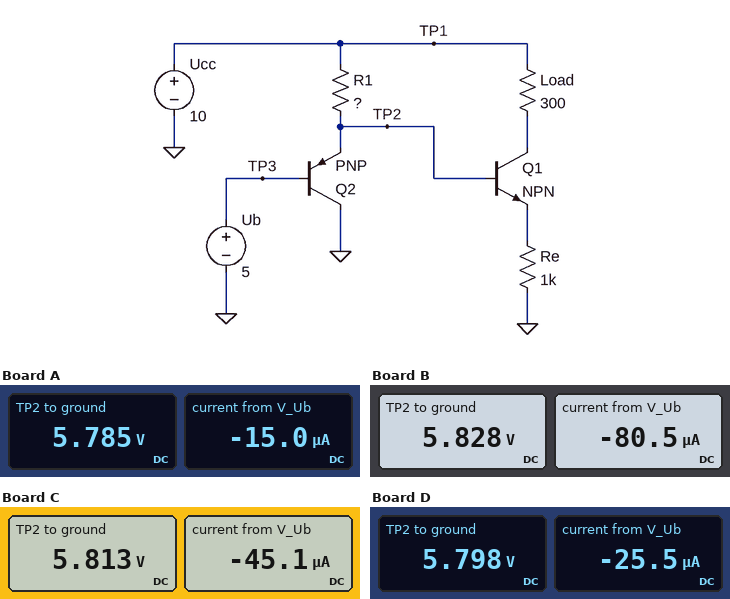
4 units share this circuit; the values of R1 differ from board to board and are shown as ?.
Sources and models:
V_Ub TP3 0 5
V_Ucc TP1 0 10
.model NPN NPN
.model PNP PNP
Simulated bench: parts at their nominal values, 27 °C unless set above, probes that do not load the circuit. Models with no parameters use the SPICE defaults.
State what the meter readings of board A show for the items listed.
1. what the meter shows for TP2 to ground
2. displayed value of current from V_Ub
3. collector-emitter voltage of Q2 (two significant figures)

5.785 V
-15.0 µA
-5.8 V
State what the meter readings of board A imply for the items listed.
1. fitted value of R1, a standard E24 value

2.7 kΩ
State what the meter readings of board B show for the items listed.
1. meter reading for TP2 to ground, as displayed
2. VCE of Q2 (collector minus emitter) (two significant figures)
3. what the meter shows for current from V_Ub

5.828 V
-5.8 V
-80.5 µA
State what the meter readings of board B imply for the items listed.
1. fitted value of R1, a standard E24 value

510 Ω
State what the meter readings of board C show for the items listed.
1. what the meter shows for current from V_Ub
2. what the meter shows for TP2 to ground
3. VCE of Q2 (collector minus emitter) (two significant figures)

-45.1 µA
5.813 V
-5.8 V
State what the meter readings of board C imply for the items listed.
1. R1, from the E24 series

910 Ω
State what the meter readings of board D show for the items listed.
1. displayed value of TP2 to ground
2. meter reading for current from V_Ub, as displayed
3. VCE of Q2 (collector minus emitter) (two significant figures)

5.798 V
-25.5 µA
-5.8 V
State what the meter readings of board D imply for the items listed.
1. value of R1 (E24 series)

1.6 kΩ
